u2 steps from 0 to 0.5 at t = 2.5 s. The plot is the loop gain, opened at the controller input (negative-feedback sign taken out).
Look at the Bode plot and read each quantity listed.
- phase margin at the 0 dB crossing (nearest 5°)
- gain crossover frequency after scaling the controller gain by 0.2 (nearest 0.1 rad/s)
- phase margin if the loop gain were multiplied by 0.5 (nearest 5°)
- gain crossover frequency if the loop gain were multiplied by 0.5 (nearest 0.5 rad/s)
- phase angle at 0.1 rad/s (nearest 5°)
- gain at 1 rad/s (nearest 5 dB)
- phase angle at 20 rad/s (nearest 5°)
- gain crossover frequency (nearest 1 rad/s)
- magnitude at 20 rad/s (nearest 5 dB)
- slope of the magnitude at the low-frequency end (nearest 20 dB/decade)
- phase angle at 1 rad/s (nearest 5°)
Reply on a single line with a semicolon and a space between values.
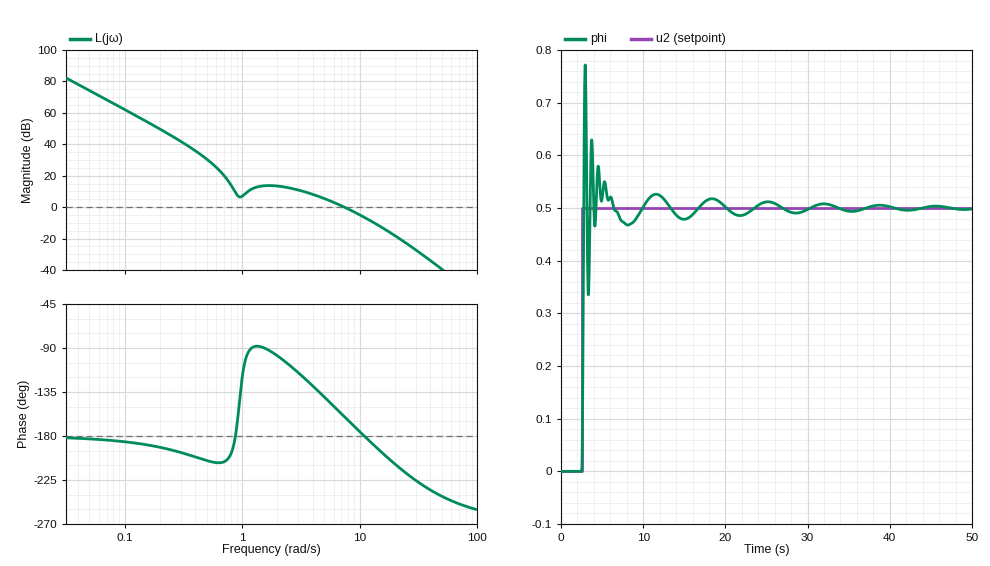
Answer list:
20°; 0.8 rad/s; 40°; 5.0 rad/s; -185°; 5 dB; -210°; 7 rad/s; -20 dB; -40 dB/decade; -120°
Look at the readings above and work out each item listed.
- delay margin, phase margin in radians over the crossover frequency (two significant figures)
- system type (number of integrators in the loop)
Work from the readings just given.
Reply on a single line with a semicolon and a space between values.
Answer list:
0.050 s; 2
